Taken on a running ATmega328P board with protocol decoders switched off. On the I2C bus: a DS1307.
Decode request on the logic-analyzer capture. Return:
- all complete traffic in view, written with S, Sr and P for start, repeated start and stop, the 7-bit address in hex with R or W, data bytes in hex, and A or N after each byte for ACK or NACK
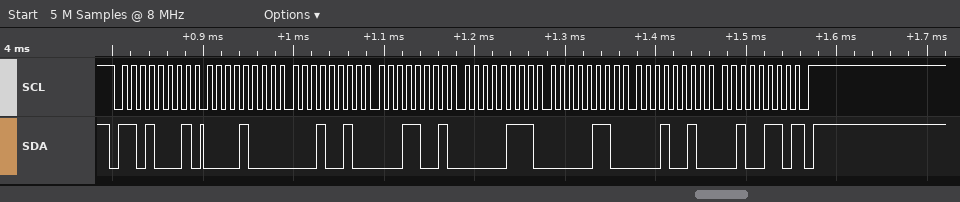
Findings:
S 68R A 08 A 12 A 19 A 07 A 06 A 12 A 26 N P
